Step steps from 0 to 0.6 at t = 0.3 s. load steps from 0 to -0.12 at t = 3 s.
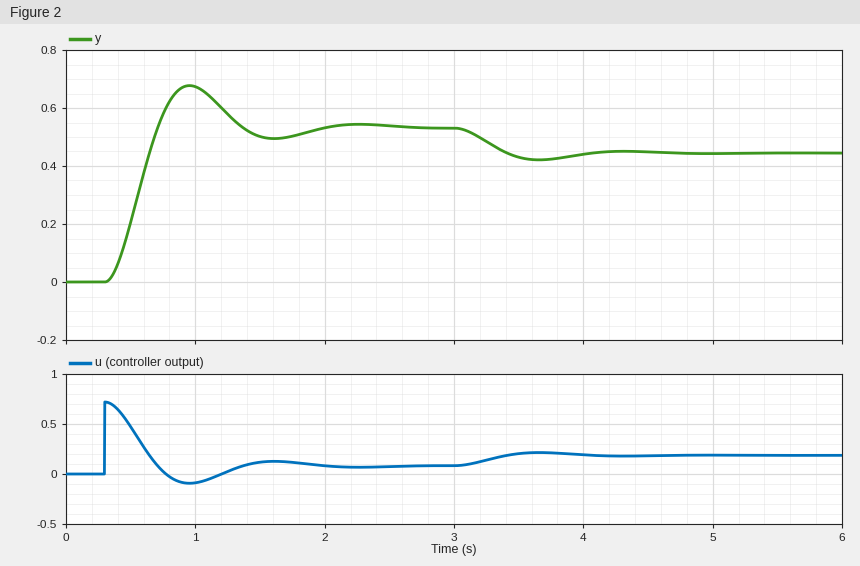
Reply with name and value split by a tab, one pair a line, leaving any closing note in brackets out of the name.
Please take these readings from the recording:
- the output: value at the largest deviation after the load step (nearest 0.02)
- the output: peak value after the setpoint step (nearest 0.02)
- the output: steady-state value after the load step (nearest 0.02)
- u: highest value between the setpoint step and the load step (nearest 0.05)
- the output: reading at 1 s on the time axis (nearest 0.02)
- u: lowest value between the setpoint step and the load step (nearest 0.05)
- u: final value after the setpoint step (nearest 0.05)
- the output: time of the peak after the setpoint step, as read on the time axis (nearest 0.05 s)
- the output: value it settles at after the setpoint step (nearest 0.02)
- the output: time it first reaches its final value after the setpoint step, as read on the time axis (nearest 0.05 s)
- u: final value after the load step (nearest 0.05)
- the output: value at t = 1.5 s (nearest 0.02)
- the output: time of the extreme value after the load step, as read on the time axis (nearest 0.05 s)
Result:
the output: value at the largest deviation after the load step	0.42
the output: peak value after the setpoint step	0.68
the output: steady-state value after the load step	0.44
u: highest value between the setpoint step and the load step	0.70
the output: reading at 1 s on the time axis	0.68
u: lowest value between the setpoint step and the load step	-0.10
u: final value after the setpoint step	0.10
the output: time of the peak after the setpoint step, as read on the time axis	0.95 s
the output: value it settles at after the setpoint step	0.54
the output: time it first reaches its final value after the setpoint step, as read on the time axis	0.70 s
u: final value after the load step	0.20
the output: value at t = 1.5 s	0.50
the output: time of the extreme value after the load step, as read on the time axis	3.65 s
